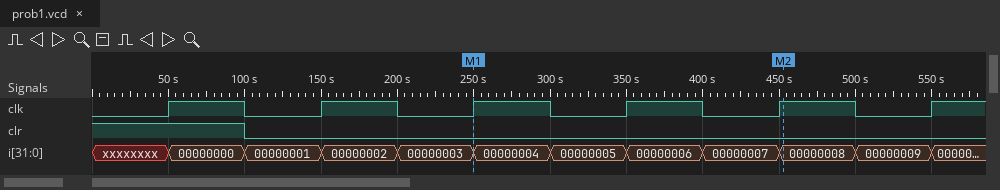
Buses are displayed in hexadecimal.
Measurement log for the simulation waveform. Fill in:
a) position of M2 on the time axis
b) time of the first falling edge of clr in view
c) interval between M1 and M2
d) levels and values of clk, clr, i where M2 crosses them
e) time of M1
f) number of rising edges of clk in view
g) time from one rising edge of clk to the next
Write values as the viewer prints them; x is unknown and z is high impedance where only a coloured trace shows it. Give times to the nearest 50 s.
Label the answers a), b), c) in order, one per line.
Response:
a) 450 s
b) 100 s
c) 200 s
d) clk=1, clr=0, i=00000008
e) 250 s
f) 6
g) 100 s
